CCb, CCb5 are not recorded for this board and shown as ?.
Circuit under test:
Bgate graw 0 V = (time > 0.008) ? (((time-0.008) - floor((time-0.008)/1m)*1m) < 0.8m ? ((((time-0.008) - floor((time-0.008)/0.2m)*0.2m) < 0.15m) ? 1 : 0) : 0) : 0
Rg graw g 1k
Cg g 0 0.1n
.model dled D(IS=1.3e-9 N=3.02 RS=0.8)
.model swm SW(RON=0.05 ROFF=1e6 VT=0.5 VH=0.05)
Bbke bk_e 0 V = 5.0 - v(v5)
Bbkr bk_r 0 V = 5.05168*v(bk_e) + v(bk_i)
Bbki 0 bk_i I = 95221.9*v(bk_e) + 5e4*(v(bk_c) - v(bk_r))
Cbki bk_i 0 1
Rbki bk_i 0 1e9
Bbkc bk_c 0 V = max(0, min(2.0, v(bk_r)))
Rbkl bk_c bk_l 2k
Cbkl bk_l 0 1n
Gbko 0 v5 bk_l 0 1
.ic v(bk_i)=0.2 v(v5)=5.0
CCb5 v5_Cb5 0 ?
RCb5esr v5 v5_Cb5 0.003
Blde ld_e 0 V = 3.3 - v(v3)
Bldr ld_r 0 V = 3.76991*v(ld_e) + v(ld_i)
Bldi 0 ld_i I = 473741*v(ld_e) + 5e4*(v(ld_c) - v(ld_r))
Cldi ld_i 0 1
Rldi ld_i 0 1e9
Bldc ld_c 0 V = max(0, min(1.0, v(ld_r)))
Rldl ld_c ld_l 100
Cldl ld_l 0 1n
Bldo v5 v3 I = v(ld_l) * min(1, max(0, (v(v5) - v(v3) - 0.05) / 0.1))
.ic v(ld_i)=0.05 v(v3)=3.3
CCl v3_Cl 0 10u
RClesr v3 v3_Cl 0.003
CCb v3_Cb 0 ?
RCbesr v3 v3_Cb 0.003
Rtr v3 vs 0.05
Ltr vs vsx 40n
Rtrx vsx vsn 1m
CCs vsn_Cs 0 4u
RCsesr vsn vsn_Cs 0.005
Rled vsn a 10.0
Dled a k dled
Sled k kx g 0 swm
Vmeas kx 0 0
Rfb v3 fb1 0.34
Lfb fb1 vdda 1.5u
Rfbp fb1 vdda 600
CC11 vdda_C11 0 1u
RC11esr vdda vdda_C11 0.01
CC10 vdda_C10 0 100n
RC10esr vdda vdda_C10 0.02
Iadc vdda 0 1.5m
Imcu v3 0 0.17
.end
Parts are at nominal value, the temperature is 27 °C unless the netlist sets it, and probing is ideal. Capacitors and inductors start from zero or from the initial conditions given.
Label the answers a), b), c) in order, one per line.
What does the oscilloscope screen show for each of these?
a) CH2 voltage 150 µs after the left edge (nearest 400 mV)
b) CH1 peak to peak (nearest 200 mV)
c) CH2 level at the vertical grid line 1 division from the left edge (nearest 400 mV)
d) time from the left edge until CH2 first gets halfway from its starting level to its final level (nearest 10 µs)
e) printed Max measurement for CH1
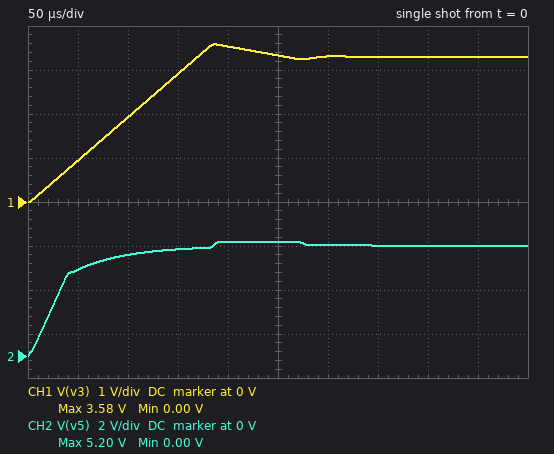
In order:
a) 4.8 V
b) 3.6 V
c) 4.0 V
d) 30 µs
e) 3.58 V
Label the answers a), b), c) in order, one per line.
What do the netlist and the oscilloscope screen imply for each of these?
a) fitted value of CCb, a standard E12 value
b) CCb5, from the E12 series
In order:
a) 27 µF
b) 10 µF
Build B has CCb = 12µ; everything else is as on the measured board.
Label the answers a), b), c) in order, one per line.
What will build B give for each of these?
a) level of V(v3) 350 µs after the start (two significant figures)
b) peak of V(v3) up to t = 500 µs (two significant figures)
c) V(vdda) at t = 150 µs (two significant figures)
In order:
a) 3.3 V
b) 3.7 V
c) 3.6 V
